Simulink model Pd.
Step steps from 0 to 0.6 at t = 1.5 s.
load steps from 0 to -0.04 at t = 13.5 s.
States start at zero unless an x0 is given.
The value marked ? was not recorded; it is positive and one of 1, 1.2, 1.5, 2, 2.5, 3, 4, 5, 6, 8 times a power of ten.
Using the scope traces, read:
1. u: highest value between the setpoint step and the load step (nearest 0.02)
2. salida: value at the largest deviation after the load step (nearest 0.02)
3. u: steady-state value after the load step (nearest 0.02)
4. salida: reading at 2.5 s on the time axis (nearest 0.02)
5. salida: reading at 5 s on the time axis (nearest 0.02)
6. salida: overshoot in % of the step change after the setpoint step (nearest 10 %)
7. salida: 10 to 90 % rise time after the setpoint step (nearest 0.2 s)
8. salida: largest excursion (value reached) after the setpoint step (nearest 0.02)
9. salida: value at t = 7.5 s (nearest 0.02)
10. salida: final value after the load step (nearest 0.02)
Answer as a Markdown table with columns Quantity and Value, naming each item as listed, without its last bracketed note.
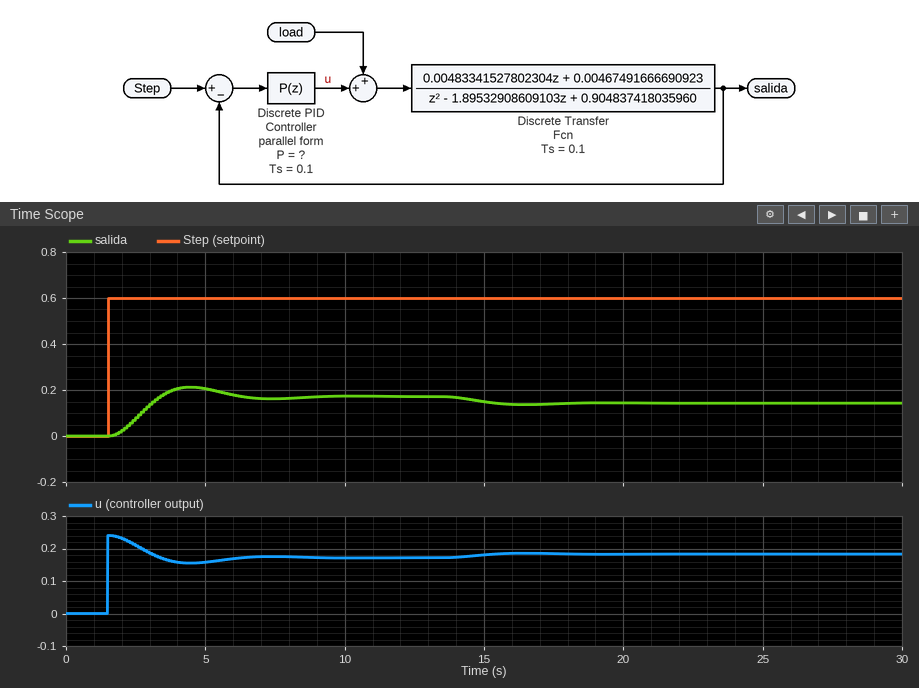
| Quantity | Value |
|---|---|
| u: highest value between the setpoint step and the load step | 0.24 |
| salida: value at the largest deviation after the load step | 0.14 |
| u: steady-state value after the load step | 0.18 |
| salida: reading at 2.5 s on the time axis | 0.08 |
| salida: reading at 5 s on the time axis | 0.20 |
| salida: overshoot in % of the step change after the setpoint step | 20 % |
| salida: 10 to 90 % rise time after the setpoint step | 1.2 s |
| salida: largest excursion (value reached) after the setpoint step | 0.22 |
| salida: value at t = 7.5 s | 0.16 |
| salida: final value after the load step | 0.14 |
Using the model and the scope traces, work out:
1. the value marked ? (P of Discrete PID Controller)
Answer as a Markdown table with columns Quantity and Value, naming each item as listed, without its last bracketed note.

| Quantity | Value |
|---|---|
| the value marked ? | 0.4 |
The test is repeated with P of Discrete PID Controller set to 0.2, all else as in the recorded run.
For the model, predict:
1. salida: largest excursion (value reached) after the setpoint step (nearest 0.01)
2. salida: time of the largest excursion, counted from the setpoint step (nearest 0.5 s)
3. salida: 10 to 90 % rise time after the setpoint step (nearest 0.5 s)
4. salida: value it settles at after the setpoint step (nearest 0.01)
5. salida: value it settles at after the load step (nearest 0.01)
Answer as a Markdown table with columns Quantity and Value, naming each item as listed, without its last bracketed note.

| Quantity | Value |
|---|---|
| salida: largest excursion (value reached) after the setpoint step | 0.12 |
| salida: time of the largest excursion, counted from the setpoint step | 3.0 s |
| salida: 10 to 90 % rise time after the setpoint step | 1.5 s |
| salida: value it settles at after the setpoint step | 0.10 |
| salida: value it settles at after the load step | 0.07 |
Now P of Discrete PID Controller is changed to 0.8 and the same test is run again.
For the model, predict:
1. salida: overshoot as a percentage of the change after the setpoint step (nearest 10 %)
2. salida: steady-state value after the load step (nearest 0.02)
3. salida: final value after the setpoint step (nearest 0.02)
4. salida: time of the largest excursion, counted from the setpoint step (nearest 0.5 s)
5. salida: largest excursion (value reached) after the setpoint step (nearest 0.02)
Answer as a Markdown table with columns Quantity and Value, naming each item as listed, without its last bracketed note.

| Quantity | Value |
|---|---|
| salida: overshoot as a percentage of the change after the setpoint step | 30 % |
| salida: steady-state value after the load step | 0.24 |
| salida: final value after the setpoint step | 0.26 |
| salida: time of the largest excursion, counted from the setpoint step | 2.5 s |
| salida: largest excursion (value reached) after the setpoint step | 0.34 |
